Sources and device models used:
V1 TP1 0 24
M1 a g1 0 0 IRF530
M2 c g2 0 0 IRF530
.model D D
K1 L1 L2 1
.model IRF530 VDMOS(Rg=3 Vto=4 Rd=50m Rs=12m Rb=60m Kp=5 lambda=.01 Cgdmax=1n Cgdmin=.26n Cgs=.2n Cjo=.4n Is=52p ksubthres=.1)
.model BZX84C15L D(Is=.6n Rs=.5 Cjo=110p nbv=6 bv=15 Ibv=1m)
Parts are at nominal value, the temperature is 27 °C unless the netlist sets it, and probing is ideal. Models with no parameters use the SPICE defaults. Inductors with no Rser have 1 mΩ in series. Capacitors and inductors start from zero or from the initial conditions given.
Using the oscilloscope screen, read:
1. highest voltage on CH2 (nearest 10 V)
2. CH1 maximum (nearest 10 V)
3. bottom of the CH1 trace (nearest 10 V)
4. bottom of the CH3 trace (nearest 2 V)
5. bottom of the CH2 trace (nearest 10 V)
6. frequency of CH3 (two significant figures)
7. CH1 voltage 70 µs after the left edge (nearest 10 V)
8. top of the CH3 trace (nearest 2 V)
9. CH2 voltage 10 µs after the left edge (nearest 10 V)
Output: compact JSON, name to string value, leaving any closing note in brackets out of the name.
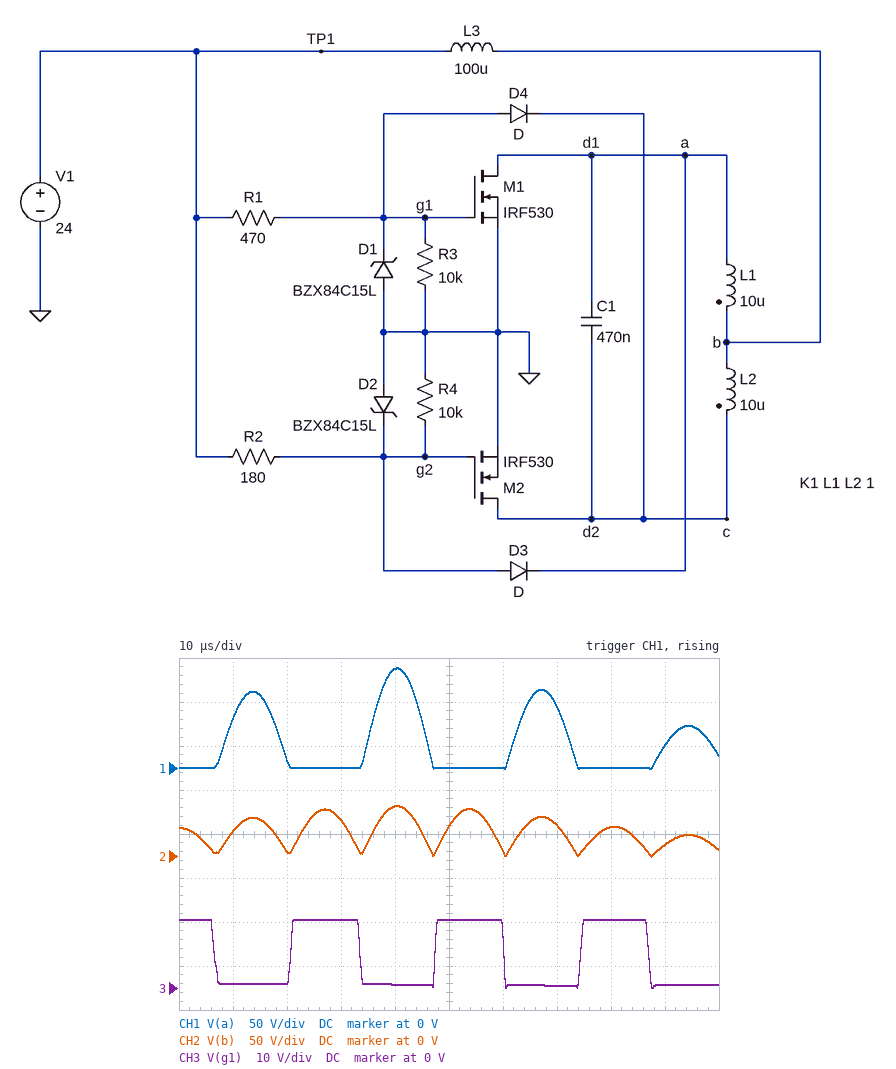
{"highest voltage on CH2": "60 V", "CH1 maximum": "110 V", "bottom of the CH1 trace": "0 V", "bottom of the CH3 trace": "0 V", "bottom of the CH2 trace": "0 V", "frequency of CH3": "37 kHz", "CH1 voltage 70 µs after the left edge": "70 V", "top of the CH3 trace": "16 V", "CH2 voltage 10 µs after the left edge": "30 V"}
